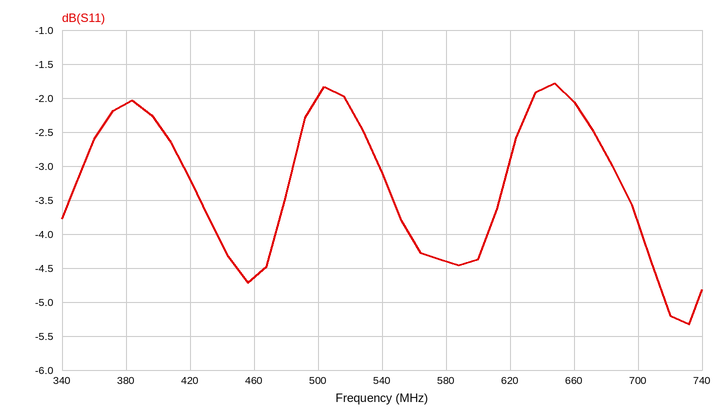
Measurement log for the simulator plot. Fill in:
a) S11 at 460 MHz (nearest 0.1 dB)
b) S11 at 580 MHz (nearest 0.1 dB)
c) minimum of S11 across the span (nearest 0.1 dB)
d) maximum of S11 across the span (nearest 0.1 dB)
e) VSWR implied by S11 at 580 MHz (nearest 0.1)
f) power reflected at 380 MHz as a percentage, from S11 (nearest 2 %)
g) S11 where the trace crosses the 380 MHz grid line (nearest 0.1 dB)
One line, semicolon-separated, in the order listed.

-4.6 dB; -4.4 dB; -5.3 dB; -1.8 dB; 4.0; 62 %; -2.1 dB
